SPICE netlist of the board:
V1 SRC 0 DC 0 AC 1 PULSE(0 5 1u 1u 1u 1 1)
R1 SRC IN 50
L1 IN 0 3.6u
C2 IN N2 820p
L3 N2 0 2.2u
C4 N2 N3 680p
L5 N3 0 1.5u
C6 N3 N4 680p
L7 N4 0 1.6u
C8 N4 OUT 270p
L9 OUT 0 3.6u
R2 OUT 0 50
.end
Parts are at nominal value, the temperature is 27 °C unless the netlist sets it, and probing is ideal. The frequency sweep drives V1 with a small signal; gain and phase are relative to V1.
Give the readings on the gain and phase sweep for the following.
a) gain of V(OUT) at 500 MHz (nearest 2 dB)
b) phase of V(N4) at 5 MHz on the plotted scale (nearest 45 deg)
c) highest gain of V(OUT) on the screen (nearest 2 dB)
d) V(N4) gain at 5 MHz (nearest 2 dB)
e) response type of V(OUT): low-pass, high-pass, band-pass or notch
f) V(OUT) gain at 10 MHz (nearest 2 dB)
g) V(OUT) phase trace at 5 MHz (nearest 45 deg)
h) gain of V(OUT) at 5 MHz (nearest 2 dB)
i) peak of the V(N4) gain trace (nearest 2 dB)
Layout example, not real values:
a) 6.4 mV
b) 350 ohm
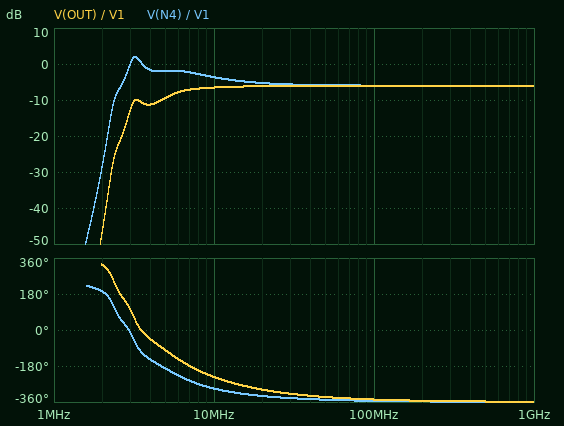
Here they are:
a) -6 dB
b) -180 deg
c) -6 dB
d) -2 dB
e) high-pass
f) -6 dB
g) -90 deg
h) -10 dB
i) 2 dB
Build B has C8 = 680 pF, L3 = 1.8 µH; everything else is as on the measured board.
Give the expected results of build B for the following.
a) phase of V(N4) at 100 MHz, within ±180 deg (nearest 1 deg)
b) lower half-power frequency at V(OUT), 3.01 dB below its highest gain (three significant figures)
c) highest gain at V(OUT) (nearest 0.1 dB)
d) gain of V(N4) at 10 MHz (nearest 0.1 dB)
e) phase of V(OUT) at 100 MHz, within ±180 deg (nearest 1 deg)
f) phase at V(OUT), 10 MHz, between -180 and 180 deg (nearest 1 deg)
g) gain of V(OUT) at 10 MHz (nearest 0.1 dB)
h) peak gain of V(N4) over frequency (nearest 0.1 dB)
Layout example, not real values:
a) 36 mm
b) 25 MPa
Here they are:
a) 8 deg
b) 2.54 MHz
c) -6.0 dB
d) -5.9 dB
e) 11 deg
f) 107 deg
g) -6.0 dB
h) -1.7 dB
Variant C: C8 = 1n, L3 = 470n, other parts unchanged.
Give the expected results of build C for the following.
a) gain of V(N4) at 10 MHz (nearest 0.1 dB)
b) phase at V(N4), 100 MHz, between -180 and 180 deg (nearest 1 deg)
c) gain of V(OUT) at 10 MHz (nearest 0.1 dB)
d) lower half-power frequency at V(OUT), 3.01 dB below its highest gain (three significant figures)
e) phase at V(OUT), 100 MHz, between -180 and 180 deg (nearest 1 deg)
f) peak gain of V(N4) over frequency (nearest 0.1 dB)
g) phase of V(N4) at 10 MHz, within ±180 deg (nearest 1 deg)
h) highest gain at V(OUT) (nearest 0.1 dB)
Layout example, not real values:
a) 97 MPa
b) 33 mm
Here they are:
a) -7.3 dB
b) 12 deg
c) -7.2 dB
d) 6.22 MHz
e) 14 deg
f) -6.0 dB
g) 114 deg
h) -6.0 dB
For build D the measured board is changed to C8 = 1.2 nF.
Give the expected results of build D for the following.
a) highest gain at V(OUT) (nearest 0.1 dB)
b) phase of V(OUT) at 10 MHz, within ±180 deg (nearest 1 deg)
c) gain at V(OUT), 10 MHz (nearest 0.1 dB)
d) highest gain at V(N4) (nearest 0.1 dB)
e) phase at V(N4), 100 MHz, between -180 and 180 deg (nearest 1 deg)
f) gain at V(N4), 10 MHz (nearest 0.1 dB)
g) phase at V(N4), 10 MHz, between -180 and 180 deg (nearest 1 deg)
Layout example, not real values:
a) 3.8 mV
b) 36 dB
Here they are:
a) -6.0 dB
b) 99 deg
c) -6.1 dB
d) -6.0 dB
e) 8 deg
f) -6.3 dB
g) 83 deg
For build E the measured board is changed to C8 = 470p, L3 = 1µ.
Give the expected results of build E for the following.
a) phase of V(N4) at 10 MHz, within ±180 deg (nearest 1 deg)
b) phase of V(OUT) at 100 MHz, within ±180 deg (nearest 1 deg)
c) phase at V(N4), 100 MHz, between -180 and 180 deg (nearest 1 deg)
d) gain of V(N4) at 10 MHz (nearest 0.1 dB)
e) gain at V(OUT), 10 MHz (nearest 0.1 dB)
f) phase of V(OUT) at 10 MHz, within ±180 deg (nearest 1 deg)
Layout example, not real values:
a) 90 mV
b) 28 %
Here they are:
a) 85 deg
b) 12 deg
c) 8 deg
d) -5.7 dB
e) -6.4 dB
f) 124 deg
